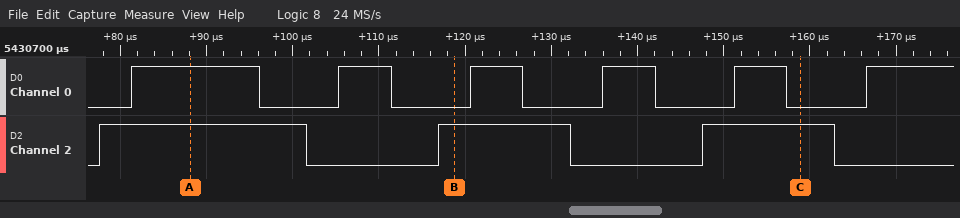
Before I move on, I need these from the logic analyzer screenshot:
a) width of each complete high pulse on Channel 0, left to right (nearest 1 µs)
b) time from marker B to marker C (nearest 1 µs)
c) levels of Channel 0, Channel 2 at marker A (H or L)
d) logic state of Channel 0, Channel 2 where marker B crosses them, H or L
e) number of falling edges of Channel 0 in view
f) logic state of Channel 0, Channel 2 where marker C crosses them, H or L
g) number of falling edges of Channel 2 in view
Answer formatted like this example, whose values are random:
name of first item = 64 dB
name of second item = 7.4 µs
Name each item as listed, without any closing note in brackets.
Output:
width of each complete high pulse on Channel 0, left to right = 15 µs, 6 µs, 6 µs, 6 µs, 6 µs
time from marker B to marker C = 40 µs
levels of Channel 0, Channel 2 at marker A = Channel 0=H, Channel 2=H
logic state of Channel 0, Channel 2 where marker B crosses them, H or L = Channel 0=L, Channel 2=H
number of falling edges of Channel 0 in view = 5
logic state of Channel 0, Channel 2 where marker C crosses them, H or L = Channel 0=L, Channel 2=H
number of falling edges of Channel 2 in view = 3
